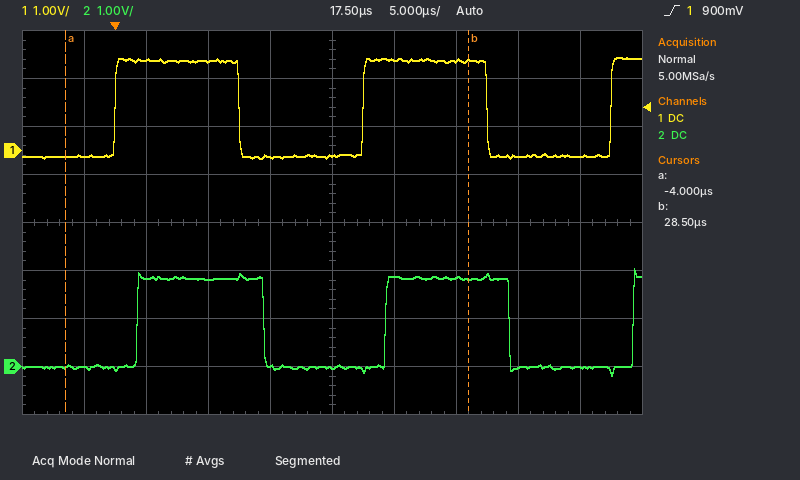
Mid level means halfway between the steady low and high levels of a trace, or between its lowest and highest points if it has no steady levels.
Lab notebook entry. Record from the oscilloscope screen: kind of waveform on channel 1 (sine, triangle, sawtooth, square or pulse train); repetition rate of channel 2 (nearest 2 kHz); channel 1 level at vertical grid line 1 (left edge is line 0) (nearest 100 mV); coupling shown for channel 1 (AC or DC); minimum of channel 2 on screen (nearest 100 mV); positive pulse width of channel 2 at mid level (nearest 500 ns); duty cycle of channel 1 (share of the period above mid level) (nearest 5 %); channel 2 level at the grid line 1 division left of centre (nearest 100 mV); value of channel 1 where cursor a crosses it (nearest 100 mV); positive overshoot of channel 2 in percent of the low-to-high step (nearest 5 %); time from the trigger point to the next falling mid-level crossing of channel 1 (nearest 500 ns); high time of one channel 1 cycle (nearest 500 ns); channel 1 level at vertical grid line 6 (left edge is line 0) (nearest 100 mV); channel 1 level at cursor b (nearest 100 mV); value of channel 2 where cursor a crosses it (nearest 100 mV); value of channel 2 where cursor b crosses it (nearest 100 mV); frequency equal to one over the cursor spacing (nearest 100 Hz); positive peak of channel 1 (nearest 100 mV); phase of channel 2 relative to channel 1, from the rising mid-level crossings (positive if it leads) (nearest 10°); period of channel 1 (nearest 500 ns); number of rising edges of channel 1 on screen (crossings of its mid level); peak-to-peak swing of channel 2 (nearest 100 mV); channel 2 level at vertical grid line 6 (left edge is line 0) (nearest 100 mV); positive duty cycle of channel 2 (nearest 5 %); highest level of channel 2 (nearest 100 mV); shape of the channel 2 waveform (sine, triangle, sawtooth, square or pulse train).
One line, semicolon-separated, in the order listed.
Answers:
square; 50 kHz; -100 mV; DC; -200 mV; 10.0 µs; 50 %; 0.0 V; -100 mV; 10 %; 10.0 µs; 10.0 µs; 1.9 V; 1.9 V; 0.0 V; 1.8 V; 30.8 kHz; 1.9 V; -30°; 20.0 µs; 3; 2.2 V; 1.9 V; 50 %; 2.0 V; square
